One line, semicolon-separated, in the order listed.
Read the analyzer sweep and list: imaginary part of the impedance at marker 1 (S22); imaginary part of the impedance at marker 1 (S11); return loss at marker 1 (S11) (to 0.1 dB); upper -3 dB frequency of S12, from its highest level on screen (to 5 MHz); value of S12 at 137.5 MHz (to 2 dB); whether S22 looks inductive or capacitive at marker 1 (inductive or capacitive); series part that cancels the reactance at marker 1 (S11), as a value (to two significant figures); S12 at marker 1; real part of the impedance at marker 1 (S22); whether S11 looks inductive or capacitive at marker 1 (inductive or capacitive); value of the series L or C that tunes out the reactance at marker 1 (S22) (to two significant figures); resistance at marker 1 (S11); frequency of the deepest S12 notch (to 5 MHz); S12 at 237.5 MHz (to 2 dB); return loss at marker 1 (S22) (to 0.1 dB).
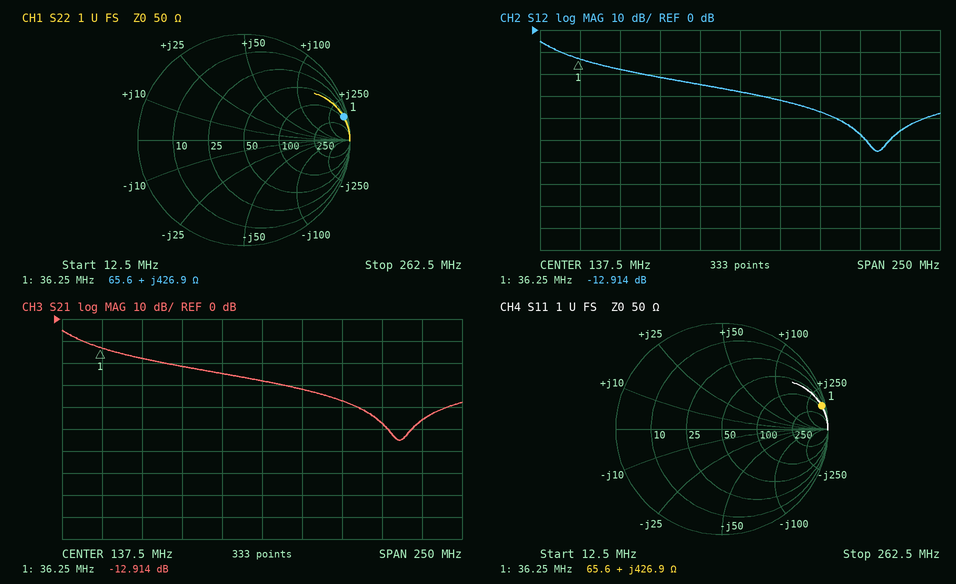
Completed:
+426.9 Ω; +426.9 Ω; 0.3 dB; 20 MHz; -28 dB; inductive; 10 pF; -12.914 dB; 65.6 Ω; inductive; 10 pF; 65.6 Ω; 225 MHz; -46 dB; 0.3 dB
